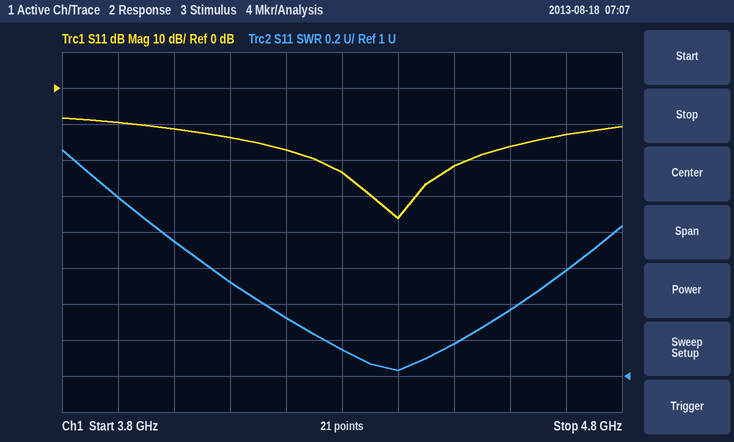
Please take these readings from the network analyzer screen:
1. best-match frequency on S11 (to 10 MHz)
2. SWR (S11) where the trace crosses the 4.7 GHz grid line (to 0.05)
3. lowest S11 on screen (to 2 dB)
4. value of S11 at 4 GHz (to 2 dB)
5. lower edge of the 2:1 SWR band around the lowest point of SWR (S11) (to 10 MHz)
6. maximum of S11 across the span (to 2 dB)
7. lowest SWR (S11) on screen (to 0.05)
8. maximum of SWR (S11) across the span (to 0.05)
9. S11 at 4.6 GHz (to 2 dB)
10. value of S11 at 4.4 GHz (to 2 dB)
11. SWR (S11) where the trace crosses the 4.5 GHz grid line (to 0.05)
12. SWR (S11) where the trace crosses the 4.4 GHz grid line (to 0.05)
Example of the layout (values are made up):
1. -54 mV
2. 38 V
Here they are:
1. 4.40 GHz
2. 1.60
3. -36 dB
4. -12 dB
5. 3.90 GHz
6. -8 dB
7. 1.05
8. 2.25
9. -16 dB
10. -36 dB
11. 1.20
12. 1.05
